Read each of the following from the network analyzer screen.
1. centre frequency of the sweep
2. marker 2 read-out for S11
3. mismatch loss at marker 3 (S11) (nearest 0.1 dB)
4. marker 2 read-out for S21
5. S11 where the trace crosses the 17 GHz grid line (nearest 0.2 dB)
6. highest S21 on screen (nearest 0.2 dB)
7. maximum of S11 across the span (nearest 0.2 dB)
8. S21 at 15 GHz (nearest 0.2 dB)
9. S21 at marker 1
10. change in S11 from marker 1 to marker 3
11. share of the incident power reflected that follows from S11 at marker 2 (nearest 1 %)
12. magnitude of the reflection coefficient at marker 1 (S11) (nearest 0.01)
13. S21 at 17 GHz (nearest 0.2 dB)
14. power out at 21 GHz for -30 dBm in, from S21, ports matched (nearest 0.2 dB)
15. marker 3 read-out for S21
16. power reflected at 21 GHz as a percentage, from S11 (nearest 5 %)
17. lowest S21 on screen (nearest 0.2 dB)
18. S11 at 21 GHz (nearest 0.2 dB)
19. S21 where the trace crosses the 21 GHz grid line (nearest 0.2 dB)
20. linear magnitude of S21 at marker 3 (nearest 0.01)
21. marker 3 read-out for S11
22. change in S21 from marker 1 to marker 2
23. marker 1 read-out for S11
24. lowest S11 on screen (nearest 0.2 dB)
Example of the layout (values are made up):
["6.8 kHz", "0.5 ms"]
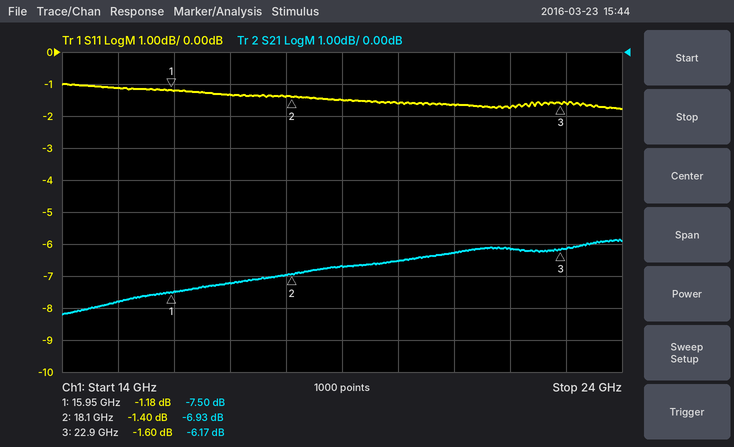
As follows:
["19 GHz", "-1.40 dB", "5.1 dB", "-6.93 dB", "-1.4 dB", "-5.8 dB", "-1.0 dB", "-7.8 dB", "-7.50 dB", "-0.42 dB", "72 %", "0.87", "-7.2 dB", "-36.2 dBm", "-6.17 dB", "70 %", "-8.2 dB", "-1.6 dB", "-6.2 dB", "0.49", "-1.60 dB", "0.57 dB", "-1.18 dB", "-1.8 dB"]
